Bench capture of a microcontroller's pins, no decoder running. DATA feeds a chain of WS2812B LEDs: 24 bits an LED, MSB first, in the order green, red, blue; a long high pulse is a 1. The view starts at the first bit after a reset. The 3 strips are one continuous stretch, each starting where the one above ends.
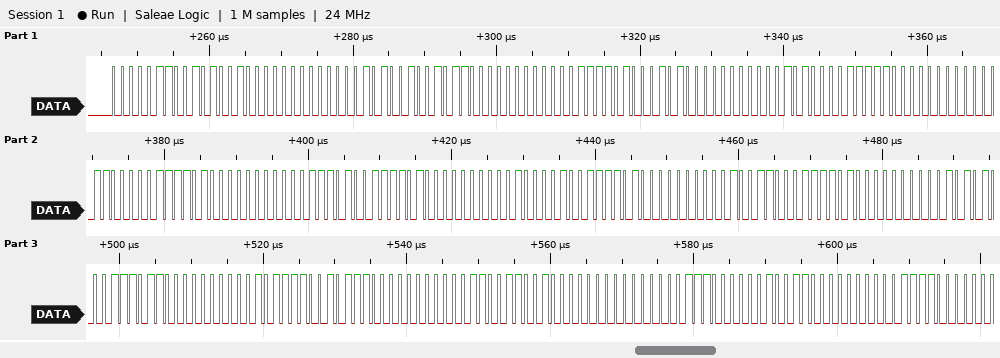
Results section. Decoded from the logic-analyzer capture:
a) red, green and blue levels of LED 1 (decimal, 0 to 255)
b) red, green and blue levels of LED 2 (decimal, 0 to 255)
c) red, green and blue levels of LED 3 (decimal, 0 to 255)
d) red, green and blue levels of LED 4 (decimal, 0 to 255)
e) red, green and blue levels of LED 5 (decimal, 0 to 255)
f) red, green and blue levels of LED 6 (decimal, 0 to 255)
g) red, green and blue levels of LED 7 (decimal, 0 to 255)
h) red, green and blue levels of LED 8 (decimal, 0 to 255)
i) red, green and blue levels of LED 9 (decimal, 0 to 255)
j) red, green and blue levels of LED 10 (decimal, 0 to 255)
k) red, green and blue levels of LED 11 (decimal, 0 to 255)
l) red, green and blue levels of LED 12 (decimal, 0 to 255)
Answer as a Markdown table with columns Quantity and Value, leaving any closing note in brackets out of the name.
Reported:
| Quantity | Value |
|---|---|
| red, green and blue levels of LED 1 | 82, 6, 0 |
| red, green and blue levels of LED 2 | 75, 10, 0 |
| red, green and blue levels of LED 3 | 69, 15, 0 |
| red, green and blue levels of LED 4 | 62, 20, 0 |
| red, green and blue levels of LED 5 | 61, 24, 0 |
| red, green and blue levels of LED 6 | 61, 29, 0 |
| red, green and blue levels of LED 7 | 61, 33, 0 |
| red, green and blue levels of LED 8 | 61, 38, 0 |
| red, green and blue levels of LED 9 | 59, 42, 0 |
| red, green and blue levels of LED 10 | 46, 47, 0 |
| red, green and blue levels of LED 11 | 32, 51, 0 |
| red, green and blue levels of LED 12 | 19, 56, 0 |
